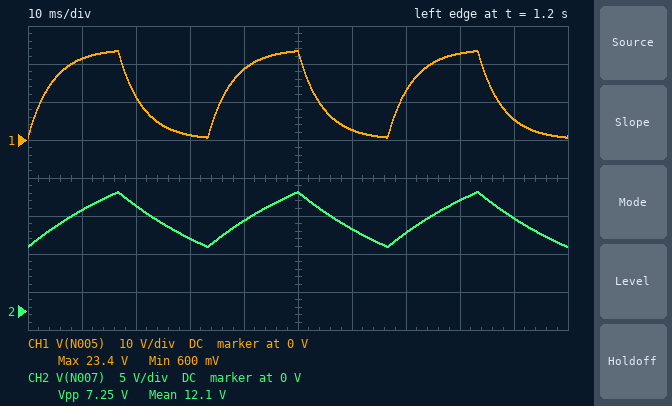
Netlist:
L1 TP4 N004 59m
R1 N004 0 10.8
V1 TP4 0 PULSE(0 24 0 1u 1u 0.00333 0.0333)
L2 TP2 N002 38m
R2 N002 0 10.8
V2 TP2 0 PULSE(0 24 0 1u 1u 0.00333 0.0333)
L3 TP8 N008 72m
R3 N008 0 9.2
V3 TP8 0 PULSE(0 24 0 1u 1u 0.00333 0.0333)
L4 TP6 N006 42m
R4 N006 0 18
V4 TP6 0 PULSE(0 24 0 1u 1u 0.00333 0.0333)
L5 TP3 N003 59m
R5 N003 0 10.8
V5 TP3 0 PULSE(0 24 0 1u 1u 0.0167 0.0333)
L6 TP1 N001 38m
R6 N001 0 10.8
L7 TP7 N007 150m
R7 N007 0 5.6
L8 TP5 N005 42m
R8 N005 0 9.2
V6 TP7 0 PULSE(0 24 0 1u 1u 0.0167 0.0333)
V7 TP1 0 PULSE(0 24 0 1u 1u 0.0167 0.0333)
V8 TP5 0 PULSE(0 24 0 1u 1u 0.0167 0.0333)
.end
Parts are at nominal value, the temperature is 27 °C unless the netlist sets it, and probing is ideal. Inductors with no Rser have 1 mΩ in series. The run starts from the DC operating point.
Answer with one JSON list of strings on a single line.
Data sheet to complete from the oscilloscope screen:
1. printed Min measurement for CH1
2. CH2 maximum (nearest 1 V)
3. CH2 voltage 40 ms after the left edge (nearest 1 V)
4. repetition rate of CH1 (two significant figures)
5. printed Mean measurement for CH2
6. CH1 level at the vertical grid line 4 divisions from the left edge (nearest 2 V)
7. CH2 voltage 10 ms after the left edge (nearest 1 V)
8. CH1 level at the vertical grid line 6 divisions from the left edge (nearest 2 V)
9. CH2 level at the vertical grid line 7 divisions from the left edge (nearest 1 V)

["600 mV", "16 V", "12 V", "30 Hz", "12.1 V", "18 V", "13 V", "2 V", "10 V"]
